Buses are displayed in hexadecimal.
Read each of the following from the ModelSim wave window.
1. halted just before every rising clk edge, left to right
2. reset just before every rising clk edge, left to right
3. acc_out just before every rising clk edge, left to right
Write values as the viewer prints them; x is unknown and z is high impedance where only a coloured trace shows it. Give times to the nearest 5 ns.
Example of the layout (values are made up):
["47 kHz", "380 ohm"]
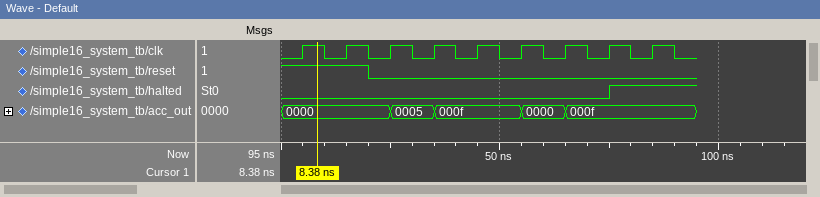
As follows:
["0 0 0 0 0 0 0 0 1", "1 1 0 0 0 0 0 0 0", "0000, 0000, 0000, 0005, 000f, 000f, 0000, 000f, 000f"]
